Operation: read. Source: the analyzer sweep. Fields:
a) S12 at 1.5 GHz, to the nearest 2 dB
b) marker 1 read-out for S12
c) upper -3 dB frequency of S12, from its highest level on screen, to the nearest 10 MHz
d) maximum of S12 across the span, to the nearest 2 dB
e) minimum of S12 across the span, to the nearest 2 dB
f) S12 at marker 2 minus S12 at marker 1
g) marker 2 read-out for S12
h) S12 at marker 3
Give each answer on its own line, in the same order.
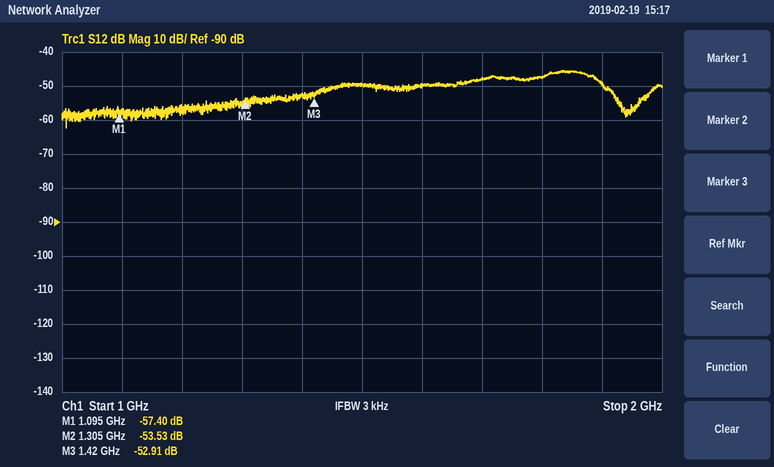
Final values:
-50 dB
-57.40 dB
1.89 GHz
-46 dB
-62 dB
3.87 dB
-53.53 dB
-52.91 dB
